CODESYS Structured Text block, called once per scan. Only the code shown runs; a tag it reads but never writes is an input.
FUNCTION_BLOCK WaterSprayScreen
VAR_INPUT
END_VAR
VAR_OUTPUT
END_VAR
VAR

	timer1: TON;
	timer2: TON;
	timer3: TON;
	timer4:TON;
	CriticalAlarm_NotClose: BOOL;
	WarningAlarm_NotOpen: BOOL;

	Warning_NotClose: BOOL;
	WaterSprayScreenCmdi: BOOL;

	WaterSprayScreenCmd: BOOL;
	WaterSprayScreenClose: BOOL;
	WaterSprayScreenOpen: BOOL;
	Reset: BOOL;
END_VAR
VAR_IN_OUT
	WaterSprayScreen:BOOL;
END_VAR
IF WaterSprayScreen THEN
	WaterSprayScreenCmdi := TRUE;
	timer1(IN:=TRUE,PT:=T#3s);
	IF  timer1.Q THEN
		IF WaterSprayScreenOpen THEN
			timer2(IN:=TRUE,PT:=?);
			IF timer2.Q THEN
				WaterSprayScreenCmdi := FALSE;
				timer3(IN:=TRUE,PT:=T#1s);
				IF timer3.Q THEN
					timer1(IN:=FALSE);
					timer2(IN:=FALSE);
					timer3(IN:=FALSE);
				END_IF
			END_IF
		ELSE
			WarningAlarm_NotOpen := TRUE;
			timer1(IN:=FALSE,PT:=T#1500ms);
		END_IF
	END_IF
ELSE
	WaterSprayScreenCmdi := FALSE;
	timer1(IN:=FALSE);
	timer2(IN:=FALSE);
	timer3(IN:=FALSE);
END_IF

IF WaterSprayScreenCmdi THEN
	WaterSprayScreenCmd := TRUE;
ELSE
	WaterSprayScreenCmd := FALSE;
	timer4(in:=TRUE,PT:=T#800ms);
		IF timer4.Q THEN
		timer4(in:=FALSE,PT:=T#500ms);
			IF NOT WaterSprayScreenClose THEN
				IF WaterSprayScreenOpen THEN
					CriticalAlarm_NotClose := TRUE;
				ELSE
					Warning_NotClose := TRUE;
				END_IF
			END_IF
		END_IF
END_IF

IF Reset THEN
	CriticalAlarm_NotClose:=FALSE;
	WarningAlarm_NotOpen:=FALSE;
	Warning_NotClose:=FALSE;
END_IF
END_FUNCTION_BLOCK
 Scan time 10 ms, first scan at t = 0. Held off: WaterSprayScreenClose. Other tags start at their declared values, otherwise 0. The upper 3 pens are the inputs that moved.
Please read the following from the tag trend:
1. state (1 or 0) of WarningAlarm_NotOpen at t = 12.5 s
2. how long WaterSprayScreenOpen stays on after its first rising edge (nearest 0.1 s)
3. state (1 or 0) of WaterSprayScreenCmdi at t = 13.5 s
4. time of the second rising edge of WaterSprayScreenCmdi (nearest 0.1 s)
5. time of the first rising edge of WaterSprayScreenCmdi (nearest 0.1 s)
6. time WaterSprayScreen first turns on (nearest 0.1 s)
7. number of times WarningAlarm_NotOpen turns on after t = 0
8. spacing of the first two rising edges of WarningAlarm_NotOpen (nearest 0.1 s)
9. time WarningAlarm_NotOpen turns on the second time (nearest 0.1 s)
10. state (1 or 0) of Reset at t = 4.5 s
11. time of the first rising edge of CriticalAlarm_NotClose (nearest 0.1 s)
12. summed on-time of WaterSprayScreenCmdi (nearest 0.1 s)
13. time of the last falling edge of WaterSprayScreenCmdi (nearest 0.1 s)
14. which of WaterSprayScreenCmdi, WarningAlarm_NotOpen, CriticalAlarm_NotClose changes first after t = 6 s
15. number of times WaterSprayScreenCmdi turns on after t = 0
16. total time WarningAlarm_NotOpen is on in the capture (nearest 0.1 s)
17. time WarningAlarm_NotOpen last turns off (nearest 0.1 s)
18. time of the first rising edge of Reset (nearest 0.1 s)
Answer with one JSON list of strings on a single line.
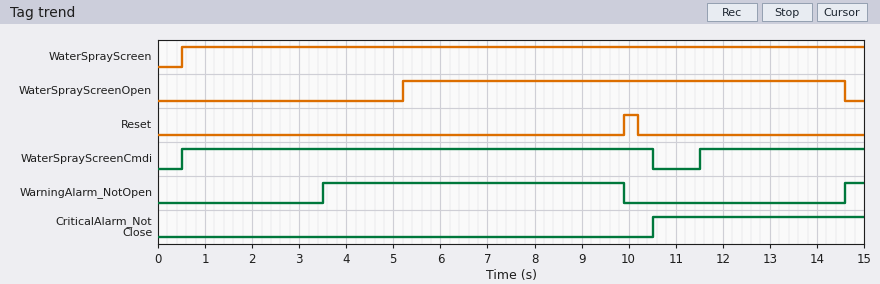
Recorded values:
["0", "9.4 s", "1", "11.5 s", "0.5 s", "0.5 s", "2", "11.1 s", "14.6 s", "0", "10.5 s", "13.5 s", "10.5 s", "WarningAlarm_NotOpen", "2", "6.8 s", "9.9 s", "9.9 s"]
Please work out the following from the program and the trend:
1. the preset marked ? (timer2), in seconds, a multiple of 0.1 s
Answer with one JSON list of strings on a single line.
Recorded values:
["4.0 s"]
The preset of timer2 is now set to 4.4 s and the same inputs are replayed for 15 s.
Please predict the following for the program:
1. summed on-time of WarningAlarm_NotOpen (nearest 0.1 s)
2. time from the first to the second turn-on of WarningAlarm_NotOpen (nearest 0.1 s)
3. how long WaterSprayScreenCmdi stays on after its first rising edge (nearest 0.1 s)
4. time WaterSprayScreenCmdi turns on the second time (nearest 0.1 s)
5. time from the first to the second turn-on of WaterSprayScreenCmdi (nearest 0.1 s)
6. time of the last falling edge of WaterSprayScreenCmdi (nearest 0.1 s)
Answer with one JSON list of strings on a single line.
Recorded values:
["6.5 s", "11.4 s", "10.4 s", "11.9 s", "11.4 s", "10.9 s"]
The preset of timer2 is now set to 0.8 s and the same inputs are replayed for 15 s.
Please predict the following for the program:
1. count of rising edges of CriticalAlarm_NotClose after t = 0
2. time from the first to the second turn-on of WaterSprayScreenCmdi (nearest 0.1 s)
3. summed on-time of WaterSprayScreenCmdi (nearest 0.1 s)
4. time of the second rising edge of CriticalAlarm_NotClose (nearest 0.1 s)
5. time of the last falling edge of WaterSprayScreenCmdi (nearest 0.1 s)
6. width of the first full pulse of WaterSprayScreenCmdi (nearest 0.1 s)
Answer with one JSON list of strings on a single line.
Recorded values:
["2", "7.8 s", "12.5 s", "12.1 s", "12.1 s", "6.8 s"]
